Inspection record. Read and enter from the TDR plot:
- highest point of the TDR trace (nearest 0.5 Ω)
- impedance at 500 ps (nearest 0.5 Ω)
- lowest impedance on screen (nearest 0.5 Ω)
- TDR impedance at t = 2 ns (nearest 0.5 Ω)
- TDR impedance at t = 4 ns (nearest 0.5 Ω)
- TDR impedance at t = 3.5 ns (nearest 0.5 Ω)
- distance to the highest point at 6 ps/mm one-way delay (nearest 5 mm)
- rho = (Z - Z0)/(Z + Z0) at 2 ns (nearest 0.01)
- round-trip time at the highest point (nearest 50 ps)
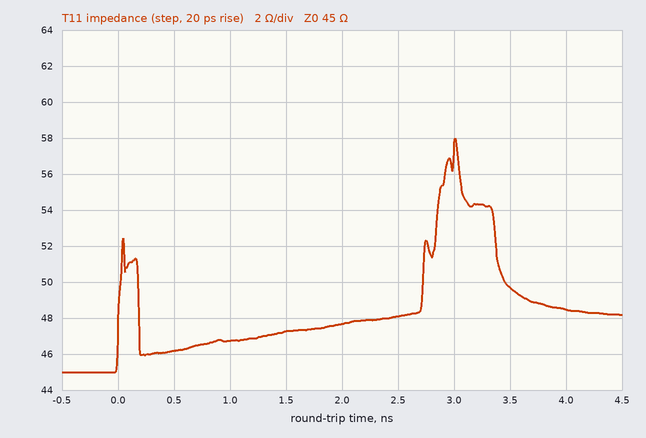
58.0 Ω
46.0 Ω
45.0 Ω
47.5 Ω
48.5 Ω
49.5 Ω
250 mm
+0.03
3.00 ns
